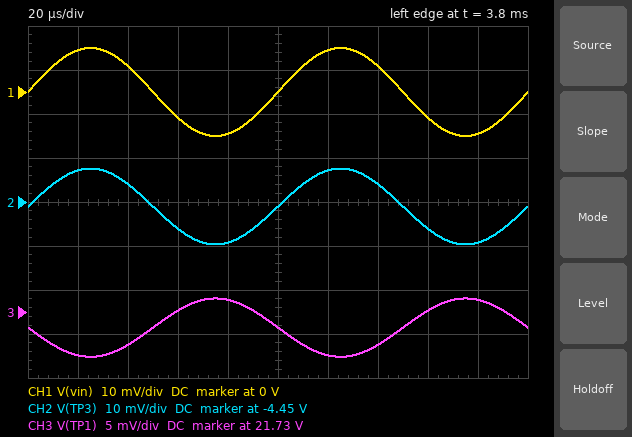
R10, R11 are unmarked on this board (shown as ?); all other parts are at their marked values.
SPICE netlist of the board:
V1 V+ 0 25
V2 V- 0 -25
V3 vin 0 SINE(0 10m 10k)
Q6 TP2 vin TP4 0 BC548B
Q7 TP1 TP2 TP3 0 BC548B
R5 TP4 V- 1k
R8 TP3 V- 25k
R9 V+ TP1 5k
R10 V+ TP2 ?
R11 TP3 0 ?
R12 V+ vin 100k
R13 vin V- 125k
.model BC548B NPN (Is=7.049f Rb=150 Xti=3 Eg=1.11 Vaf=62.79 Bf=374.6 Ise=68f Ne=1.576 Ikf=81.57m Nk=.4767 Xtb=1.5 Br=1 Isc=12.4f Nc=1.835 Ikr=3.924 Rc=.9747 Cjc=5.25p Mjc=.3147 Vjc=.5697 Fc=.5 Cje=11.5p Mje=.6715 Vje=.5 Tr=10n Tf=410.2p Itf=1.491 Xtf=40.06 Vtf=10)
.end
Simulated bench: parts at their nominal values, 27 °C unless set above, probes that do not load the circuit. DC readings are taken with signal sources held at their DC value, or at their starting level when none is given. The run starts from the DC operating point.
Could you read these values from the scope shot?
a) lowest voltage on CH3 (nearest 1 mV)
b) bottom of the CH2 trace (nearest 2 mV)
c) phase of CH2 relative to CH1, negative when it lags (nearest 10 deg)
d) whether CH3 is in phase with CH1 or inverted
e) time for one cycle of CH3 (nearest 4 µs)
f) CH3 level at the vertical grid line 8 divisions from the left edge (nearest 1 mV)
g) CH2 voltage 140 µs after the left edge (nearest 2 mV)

21.720 V
-4.460 V
0 deg
inverted
100 µs
21.725 V
-4.446 V
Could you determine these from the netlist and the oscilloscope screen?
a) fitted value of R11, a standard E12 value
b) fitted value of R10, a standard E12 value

27 kΩ
39 kΩ
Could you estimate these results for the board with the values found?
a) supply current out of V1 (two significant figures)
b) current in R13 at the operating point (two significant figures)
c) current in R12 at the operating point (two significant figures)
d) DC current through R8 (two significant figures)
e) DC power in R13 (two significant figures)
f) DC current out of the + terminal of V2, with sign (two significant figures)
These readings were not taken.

1.6 mA
200 µA
250 µA
820 µA
5.0 mW
-22 mA
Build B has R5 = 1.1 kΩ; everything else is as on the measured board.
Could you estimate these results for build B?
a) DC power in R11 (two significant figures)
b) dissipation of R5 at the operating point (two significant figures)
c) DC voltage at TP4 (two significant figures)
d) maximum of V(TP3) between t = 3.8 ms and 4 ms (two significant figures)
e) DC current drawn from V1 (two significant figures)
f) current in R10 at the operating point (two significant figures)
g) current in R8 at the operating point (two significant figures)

650 µW
420 mW
-3.6 V
-4.2 V
1.7 mA
730 µA
830 µA
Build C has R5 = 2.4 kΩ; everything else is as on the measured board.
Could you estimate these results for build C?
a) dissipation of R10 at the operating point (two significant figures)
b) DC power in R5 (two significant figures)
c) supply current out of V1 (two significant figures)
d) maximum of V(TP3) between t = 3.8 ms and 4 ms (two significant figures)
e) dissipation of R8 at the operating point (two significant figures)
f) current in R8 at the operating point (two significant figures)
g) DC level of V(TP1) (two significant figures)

19 mW
220 mW
1.7 mA
-2.7 V
20 mW
890 µA
21 V
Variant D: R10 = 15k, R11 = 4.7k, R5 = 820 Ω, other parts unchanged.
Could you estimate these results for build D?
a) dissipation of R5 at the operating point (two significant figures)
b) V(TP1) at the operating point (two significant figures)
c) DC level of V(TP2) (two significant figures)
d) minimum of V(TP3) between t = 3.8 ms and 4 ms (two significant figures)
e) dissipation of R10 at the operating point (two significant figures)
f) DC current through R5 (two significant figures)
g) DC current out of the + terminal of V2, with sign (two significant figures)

520 mW
25 V
-4.2 V
-4.0 V
57 mW
25 mA
-26 mA
